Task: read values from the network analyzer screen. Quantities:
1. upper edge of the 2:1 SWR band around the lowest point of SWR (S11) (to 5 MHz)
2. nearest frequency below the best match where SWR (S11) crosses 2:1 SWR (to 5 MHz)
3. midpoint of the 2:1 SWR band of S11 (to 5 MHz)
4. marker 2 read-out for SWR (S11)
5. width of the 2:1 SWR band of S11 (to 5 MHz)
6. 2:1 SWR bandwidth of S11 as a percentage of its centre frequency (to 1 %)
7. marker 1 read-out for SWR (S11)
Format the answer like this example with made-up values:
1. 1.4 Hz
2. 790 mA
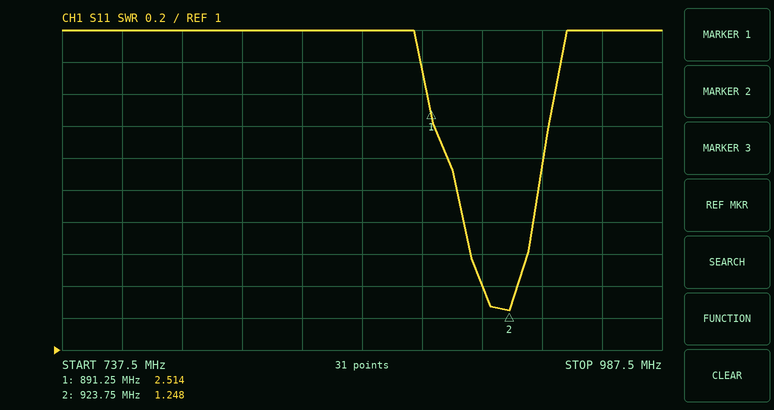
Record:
1. 935 MHz
2. 900 MHz
3. 920 MHz
4. 1.248
5. 35 MHz
6. 4 %
7. 2.514
